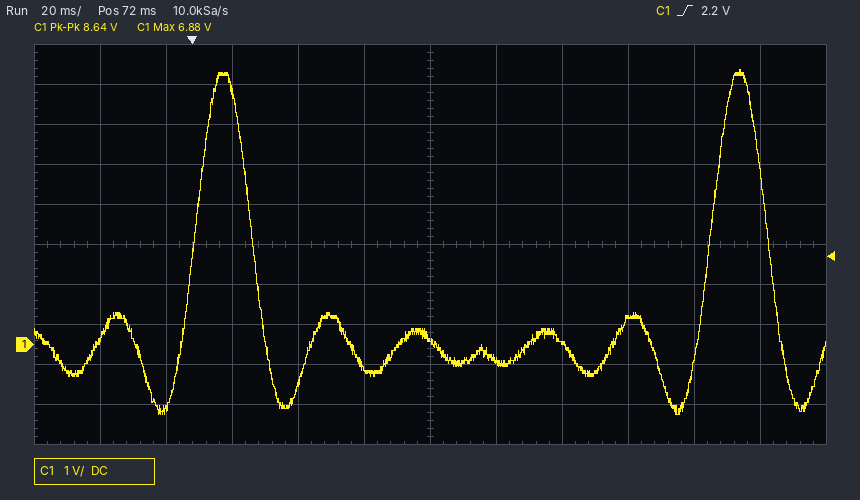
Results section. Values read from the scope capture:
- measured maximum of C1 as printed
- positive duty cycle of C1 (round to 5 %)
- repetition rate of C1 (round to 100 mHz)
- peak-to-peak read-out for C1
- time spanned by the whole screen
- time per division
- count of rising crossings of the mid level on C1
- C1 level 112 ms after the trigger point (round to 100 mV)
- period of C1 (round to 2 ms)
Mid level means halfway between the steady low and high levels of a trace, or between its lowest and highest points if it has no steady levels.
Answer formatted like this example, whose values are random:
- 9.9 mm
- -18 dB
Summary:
- 6.88 V
- 10 %
- 6.4 Hz
- 8.64 V
- 240 ms
- 20 ms
- 2
- 0.0 V
- 156 ms
